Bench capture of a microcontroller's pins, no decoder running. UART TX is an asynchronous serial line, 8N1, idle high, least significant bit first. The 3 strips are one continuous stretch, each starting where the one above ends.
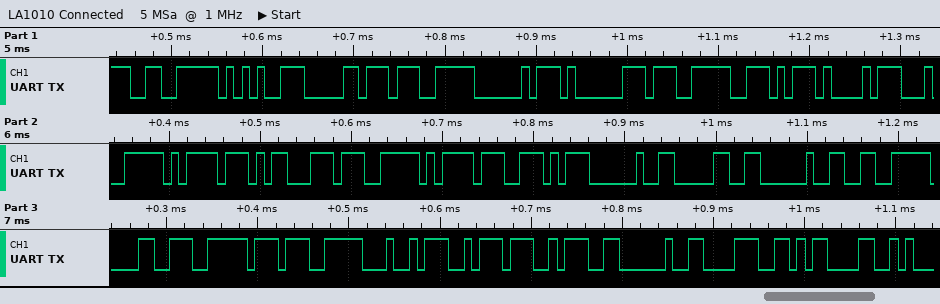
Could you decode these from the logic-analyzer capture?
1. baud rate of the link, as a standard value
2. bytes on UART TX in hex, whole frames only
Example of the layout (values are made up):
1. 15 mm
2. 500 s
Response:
1. 115200 baud
2. E6 95 B0 E7 A0 81 E7 AE A1 E4 BD 8D E7 BD AE 20 30 20 E6 98 BE E7 A4 BA 3A 20 38 0D
